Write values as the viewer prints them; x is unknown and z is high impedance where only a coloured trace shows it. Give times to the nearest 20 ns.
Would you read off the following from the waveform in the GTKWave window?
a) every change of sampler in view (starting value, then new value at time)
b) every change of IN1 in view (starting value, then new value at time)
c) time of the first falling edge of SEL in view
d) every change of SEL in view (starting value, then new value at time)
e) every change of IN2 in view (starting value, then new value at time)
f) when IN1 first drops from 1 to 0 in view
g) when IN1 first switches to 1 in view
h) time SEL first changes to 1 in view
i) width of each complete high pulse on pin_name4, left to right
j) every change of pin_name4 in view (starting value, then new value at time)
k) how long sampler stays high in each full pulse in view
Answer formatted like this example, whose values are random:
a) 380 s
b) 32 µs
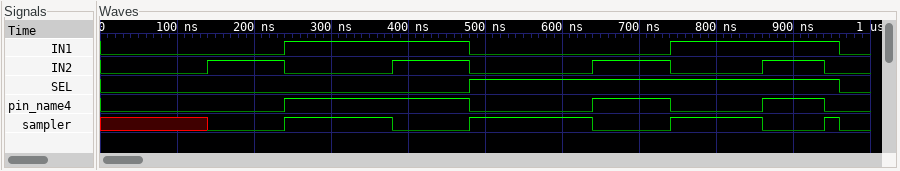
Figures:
a) x, 0 at 140 ns, 1 at 240 ns, 0 at 380 ns, 1 at 480 ns, 0 at 640 ns, 1 at 740 ns, 0 at 860 ns, 1 at 940 ns, 0 at 960 ns
b) 0, 1 at 240 ns, 0 at 480 ns, 1 at 740 ns, 0 at 960 ns
c) 960 ns
d) 0, 1 at 480 ns, 0 at 960 ns
e) 0, 1 at 140 ns, 0 at 240 ns, 1 at 380 ns, 0 at 480 ns, 1 at 640 ns, 0 at 740 ns, 1 at 860 ns, 0 at 940 ns
f) 480 ns
g) 240 ns
h) 480 ns
i) 240 ns, 100 ns, 80 ns
j) 0, 1 at 240 ns, 0 at 480 ns, 1 at 640 ns, 0 at 740 ns, 1 at 860 ns, 0 at 940 ns
k) 140 ns, 160 ns, 120 ns, 20 ns
